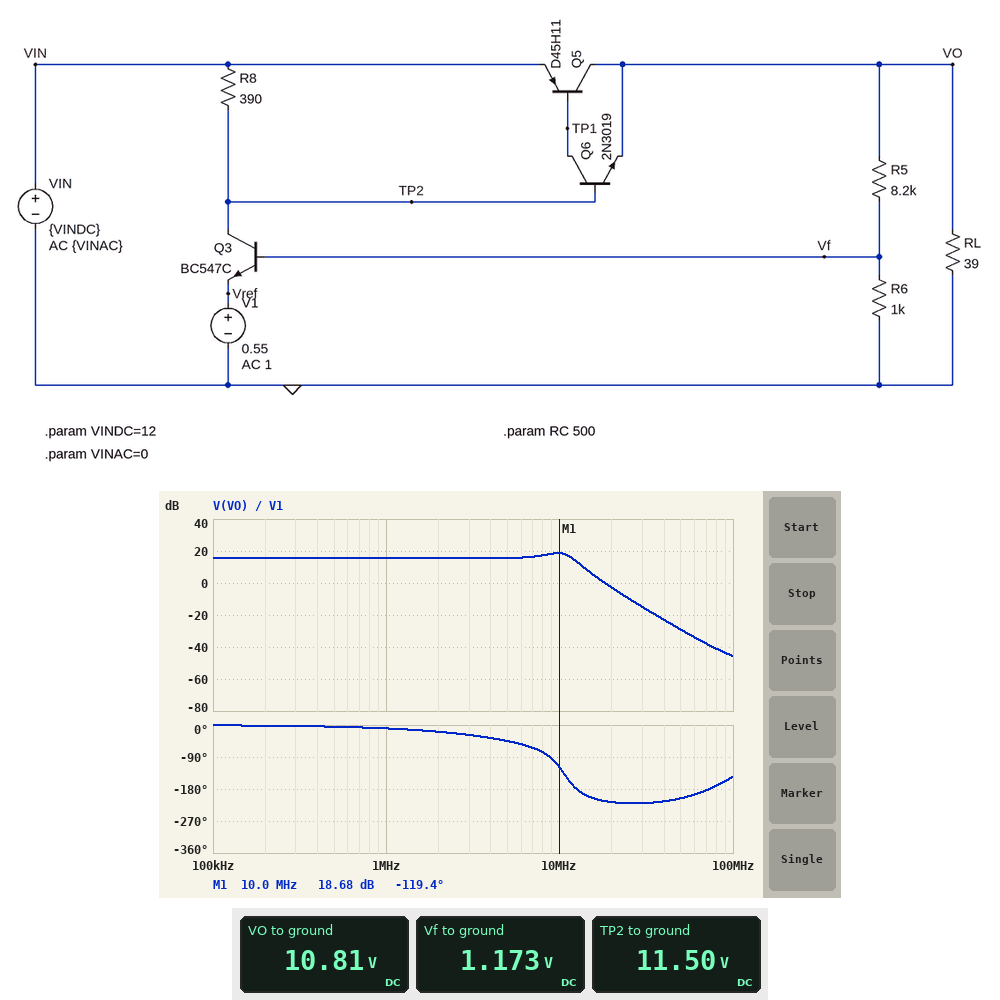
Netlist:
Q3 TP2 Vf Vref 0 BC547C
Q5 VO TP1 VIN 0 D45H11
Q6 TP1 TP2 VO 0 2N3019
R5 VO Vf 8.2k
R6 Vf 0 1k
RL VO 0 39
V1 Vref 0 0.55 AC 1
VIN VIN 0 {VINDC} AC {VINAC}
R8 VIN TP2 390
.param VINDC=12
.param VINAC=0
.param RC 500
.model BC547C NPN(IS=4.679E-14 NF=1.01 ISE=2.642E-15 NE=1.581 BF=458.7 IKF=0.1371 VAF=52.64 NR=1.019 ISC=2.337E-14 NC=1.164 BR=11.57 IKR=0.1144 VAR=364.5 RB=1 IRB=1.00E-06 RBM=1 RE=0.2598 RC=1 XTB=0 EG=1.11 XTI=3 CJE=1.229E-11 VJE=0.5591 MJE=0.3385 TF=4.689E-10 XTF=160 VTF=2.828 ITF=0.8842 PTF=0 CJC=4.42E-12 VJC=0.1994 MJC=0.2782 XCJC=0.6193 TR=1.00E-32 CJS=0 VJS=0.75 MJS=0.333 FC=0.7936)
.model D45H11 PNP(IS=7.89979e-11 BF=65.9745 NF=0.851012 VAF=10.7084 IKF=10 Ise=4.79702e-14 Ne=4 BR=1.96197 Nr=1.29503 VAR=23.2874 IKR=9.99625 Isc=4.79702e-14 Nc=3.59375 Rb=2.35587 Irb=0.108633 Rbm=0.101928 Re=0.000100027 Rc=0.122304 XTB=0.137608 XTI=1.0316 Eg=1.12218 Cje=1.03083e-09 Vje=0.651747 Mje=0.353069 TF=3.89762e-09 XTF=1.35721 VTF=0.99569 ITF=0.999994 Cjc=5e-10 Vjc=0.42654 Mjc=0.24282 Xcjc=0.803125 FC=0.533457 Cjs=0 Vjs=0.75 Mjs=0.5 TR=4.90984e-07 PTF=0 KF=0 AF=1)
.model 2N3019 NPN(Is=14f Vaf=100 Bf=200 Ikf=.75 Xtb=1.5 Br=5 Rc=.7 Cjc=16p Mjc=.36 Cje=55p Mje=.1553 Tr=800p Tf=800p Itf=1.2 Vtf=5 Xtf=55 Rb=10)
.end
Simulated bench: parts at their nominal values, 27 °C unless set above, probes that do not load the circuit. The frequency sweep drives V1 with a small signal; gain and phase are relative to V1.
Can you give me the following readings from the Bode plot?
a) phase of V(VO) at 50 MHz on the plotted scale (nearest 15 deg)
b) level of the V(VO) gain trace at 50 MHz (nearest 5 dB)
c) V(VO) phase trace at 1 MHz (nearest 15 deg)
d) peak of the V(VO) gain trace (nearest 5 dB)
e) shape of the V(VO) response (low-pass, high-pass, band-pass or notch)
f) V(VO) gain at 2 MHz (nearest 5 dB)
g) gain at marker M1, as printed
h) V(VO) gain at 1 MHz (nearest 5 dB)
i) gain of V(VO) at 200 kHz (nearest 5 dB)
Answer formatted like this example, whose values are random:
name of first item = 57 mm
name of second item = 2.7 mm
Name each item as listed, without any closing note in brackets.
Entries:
phase of V(VO) at 50 MHz on the plotted scale = -210 deg
level of the V(VO) gain trace at 50 MHz = -30 dB
V(VO) phase trace at 1 MHz = -15 deg
peak of the V(VO) gain trace = 20 dB
shape of the V(VO) response = low-pass
V(VO) gain at 2 MHz = 15 dB
gain at marker M1, as printed = 18.68 dB
V(VO) gain at 1 MHz = 15 dB
gain of V(VO) at 200 kHz = 15 dB
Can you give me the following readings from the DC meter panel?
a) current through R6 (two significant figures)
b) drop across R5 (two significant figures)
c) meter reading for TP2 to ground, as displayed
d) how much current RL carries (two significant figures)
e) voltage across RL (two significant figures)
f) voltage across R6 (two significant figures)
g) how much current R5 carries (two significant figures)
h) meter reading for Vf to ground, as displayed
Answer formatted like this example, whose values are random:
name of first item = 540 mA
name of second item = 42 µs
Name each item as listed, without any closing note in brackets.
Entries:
current through R6 = 1.2 mA
drop across R5 = 9.6 V
meter reading for TP2 to ground, as displayed = 11.50 V
how much current RL carries = 280 mA
voltage across RL = 11 V
voltage across R6 = 1.2 V
how much current R5 carries = 1.2 mA
meter reading for Vf to ground, as displayed = 1.173 V
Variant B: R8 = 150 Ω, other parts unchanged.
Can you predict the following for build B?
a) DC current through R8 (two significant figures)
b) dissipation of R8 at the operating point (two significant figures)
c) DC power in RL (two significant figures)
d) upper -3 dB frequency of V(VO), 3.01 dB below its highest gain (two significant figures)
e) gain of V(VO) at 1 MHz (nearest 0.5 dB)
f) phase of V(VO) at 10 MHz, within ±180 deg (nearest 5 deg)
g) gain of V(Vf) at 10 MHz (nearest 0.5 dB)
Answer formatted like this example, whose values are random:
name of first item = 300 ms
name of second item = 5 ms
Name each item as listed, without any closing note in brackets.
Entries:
DC current through R8 = 2.3 mA
dissipation of R8 at the operating point = 780 µW
DC power in RL = 3.1 W
upper -3 dB frequency of V(VO), 3.01 dB below its highest gain = 7.6 MHz
gain of V(VO) at 1 MHz = 14.0 dB
phase of V(VO) at 10 MHz, within ±180 deg = -90 deg
gain of V(Vf) at 10 MHz = -1.0 dB
